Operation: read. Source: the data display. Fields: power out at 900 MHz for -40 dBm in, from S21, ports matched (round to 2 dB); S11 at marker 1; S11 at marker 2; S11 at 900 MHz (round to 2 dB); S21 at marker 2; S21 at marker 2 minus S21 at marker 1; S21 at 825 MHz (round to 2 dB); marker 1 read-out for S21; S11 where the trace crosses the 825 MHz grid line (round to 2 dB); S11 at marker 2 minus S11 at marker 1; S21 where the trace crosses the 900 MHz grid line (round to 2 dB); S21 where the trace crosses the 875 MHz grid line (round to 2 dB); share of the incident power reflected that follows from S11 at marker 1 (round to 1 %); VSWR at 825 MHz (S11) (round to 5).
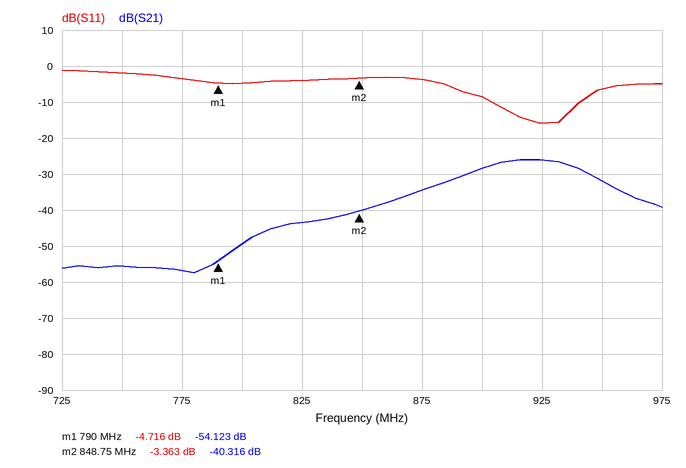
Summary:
-68 dBm
-4.716 dB
-3.363 dB
-8 dB
-40.316 dB
13.807 dB
-44 dB
-54.123 dB
-4 dB
1.353 dB
-28 dB
-34 dB
34 %
5
